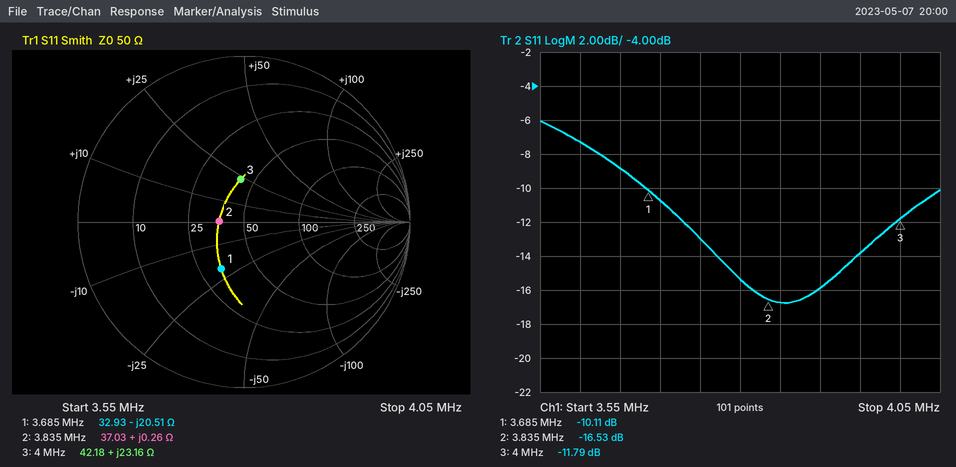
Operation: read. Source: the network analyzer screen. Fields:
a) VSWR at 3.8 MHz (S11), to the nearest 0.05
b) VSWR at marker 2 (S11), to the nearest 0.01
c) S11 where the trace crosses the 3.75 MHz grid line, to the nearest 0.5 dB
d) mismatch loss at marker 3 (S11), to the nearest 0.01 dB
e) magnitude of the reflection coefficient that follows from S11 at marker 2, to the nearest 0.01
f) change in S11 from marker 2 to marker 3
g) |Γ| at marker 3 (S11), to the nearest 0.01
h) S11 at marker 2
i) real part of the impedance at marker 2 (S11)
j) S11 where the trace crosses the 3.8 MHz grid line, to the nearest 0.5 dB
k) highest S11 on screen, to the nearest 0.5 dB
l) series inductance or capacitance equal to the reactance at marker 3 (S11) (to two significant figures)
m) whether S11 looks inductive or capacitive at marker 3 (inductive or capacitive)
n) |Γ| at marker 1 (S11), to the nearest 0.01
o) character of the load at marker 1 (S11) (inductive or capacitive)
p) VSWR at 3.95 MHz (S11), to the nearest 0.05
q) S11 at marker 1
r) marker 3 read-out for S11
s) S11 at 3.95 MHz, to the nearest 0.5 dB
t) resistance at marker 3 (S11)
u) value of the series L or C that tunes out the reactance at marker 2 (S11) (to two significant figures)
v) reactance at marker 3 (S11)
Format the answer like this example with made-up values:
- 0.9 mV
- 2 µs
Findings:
- 1.40
- 1.35
- -13.0 dB
- 0.30 dB
- 0.15
- 4.74 dB
- 0.26
- -16.53 dB
- 37.03 Ω
- -15.5 dB
- -6.0 dB
- 920 nH
- inductive
- 0.31
- capacitive
- 1.50
- -10.11 dB
- -11.79 dB
- -14.0 dB
- 42.18 Ω
- 160 nF
- +23.16 Ω
